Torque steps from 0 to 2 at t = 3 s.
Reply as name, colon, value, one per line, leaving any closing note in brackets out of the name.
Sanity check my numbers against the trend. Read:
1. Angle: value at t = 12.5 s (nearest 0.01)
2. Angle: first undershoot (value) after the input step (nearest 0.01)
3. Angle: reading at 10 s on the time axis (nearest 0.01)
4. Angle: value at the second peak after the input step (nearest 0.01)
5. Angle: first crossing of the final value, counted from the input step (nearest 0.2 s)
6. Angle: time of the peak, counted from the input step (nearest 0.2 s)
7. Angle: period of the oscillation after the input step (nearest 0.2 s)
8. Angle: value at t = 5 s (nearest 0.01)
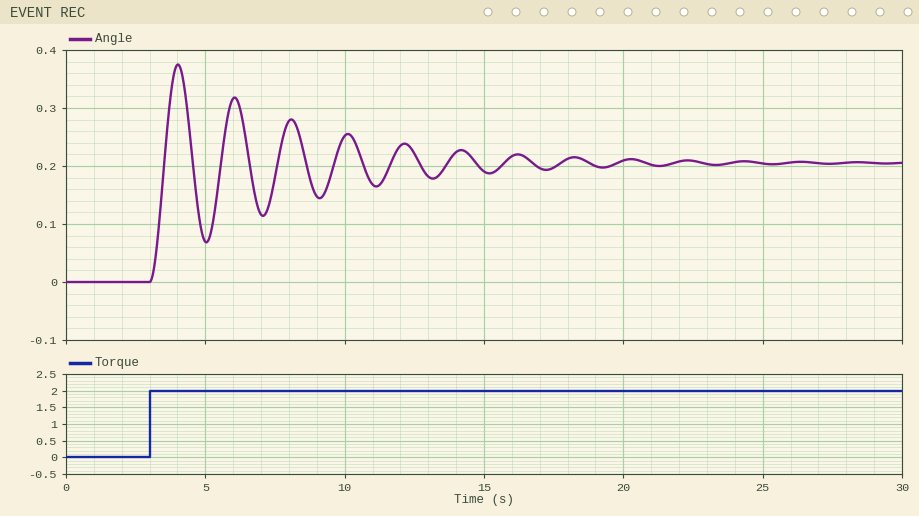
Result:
Angle: value at t = 12.5 s: 0.22
Angle: first undershoot (value) after the input step: 0.07
Angle: reading at 10 s on the time axis: 0.25
Angle: value at the second peak after the input step: 0.32
Angle: first crossing of the final value, counted from the input step: 0.6 s
Angle: time of the peak, counted from the input step: 1.0 s
Angle: period of the oscillation after the input step: 2.0 s
Angle: value at t = 5 s: 0.07
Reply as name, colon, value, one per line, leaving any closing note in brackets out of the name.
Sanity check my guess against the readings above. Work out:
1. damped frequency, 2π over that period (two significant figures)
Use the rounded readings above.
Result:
damped frequency, 2π over that period: 3.1 rad/s
